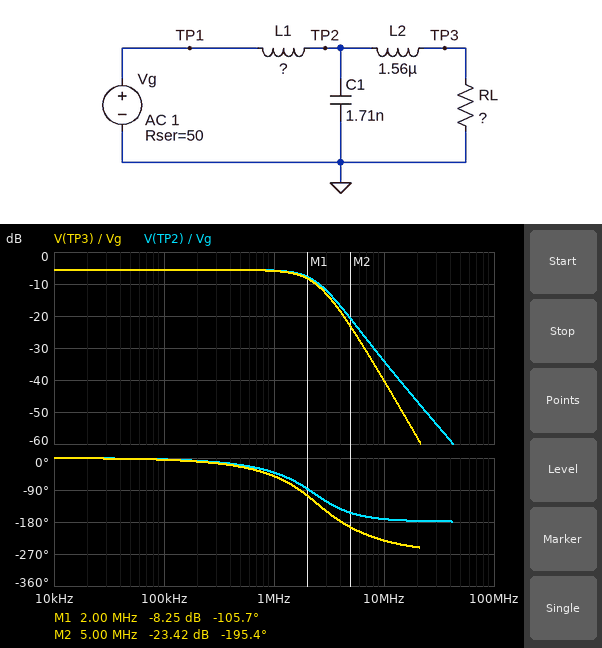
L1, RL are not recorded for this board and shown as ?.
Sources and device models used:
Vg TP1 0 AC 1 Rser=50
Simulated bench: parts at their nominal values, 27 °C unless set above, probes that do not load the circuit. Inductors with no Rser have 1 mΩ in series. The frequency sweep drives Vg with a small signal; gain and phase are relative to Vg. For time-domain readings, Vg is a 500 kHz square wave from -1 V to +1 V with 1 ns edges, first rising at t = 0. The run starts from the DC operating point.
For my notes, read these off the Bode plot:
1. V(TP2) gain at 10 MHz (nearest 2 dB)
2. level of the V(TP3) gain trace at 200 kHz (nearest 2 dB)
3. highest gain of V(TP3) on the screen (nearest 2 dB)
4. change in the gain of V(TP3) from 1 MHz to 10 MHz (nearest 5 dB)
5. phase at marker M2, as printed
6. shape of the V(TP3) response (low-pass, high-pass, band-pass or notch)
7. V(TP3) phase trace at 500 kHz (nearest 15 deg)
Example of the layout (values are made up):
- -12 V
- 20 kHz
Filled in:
- -34 dB
- -6 dB
- -6 dB
- -35 dB
- -195.4 deg
- low-pass
- -30 deg
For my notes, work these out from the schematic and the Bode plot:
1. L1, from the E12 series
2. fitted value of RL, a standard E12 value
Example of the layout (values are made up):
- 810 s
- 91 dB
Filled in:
- 8.2 µH
- 56 Ω
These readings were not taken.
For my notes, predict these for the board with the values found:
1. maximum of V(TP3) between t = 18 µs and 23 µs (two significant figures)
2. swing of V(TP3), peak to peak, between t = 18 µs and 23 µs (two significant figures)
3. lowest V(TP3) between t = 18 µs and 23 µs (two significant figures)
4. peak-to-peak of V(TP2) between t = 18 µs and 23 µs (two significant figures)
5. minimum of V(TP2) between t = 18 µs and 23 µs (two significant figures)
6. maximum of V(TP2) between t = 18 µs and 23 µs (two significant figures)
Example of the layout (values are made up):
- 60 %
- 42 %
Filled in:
- 570 mV
- 1.1 V
- -570 mV
- 1.1 V
- -570 mV
- 570 mV
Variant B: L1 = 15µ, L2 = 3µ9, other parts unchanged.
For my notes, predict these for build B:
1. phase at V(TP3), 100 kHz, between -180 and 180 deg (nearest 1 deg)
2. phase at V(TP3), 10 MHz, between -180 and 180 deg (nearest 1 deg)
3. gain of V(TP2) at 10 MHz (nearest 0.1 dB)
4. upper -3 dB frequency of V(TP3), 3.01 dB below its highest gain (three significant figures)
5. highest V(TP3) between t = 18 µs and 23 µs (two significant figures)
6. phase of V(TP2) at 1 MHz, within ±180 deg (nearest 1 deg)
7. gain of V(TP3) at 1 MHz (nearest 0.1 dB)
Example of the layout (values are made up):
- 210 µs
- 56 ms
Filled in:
- -8 deg
- 106 deg
- -39.7 dB
- 1.52 MHz
- 530 mV
- -50 deg
- -7.3 dB
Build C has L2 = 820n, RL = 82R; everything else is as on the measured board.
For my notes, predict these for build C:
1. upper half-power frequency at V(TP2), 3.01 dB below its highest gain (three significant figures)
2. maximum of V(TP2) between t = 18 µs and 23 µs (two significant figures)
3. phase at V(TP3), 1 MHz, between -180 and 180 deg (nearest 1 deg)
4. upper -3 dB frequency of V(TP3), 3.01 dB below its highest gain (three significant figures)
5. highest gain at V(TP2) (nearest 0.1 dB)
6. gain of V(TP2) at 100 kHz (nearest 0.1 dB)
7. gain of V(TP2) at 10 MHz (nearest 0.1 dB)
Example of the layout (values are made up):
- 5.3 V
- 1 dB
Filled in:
- 1.95 MHz
- 730 mV
- -49 deg
- 1.94 MHz
- -3.9 dB
- -4.1 dB
- -34.3 dB
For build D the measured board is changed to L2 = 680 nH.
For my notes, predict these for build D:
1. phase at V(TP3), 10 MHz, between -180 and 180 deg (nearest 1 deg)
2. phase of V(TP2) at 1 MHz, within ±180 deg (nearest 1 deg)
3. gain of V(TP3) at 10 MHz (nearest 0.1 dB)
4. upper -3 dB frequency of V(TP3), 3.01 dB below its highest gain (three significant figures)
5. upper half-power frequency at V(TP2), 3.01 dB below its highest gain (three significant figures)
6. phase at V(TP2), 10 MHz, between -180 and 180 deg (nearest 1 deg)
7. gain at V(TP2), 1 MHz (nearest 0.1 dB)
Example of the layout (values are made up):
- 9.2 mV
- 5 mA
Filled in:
- 155 deg
- -45 deg
- -36.1 dB
- 1.93 MHz
- 1.95 MHz
- -168 deg
- -5.9 dB
